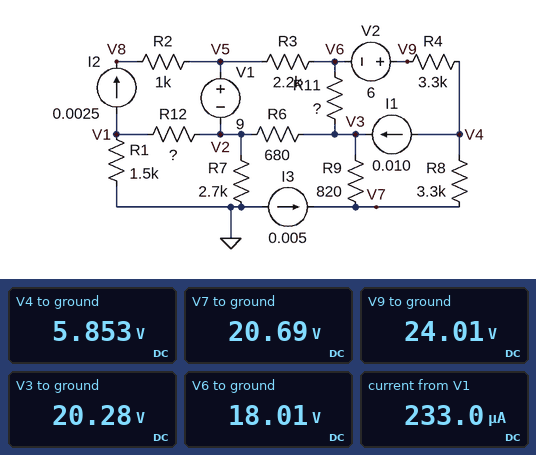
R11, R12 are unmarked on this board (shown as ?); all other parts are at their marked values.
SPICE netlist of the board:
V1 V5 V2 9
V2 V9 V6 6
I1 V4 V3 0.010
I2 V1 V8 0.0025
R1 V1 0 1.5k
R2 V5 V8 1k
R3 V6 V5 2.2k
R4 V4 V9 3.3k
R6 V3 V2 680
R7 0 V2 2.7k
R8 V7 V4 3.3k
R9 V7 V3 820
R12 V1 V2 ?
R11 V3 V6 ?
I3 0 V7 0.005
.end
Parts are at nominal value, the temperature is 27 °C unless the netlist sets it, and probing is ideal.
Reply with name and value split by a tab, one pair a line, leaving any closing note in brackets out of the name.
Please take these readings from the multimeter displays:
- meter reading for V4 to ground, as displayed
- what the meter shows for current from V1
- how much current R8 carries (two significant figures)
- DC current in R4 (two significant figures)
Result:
meter reading for V4 to ground, as displayed	5.853 V
what the meter shows for current from V1	233.0 µA
how much current R8 carries	4.5 mA
DC current in R4	5.5 mA
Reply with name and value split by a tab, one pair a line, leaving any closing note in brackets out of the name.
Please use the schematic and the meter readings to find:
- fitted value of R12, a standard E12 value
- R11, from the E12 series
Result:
fitted value of R12, a standard E12 value	8.2 kΩ
R11, from the E12 series	820 Ω
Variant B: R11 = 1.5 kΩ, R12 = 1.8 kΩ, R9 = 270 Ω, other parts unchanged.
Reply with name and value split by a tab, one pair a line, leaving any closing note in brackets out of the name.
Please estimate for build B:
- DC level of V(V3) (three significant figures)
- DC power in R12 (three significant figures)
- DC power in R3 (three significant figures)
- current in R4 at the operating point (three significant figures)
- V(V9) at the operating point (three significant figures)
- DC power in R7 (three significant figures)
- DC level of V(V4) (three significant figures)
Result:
DC level of V(V3)	15.0 V
DC power in R12	28.8 mW
DC power in R3	21.4 mW
current in R4 at the operating point	5.38 mA
V(V9) at the operating point	17.6 V
DC power in R7	33.1 mW
DC level of V(V4)	-171 mV
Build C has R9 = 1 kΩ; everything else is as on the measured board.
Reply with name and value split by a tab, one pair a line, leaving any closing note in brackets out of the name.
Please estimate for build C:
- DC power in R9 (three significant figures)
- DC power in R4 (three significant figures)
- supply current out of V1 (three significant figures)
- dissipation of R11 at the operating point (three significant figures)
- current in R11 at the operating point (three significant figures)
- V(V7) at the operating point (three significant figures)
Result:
DC power in R9	242 µW
DC power in R4	99.5 mW
supply current out of V1	231 µA
dissipation of R11 at the operating point	6.25 mW
current in R11 at the operating point	2.76 mA
V(V7) at the operating point	20.8 V
